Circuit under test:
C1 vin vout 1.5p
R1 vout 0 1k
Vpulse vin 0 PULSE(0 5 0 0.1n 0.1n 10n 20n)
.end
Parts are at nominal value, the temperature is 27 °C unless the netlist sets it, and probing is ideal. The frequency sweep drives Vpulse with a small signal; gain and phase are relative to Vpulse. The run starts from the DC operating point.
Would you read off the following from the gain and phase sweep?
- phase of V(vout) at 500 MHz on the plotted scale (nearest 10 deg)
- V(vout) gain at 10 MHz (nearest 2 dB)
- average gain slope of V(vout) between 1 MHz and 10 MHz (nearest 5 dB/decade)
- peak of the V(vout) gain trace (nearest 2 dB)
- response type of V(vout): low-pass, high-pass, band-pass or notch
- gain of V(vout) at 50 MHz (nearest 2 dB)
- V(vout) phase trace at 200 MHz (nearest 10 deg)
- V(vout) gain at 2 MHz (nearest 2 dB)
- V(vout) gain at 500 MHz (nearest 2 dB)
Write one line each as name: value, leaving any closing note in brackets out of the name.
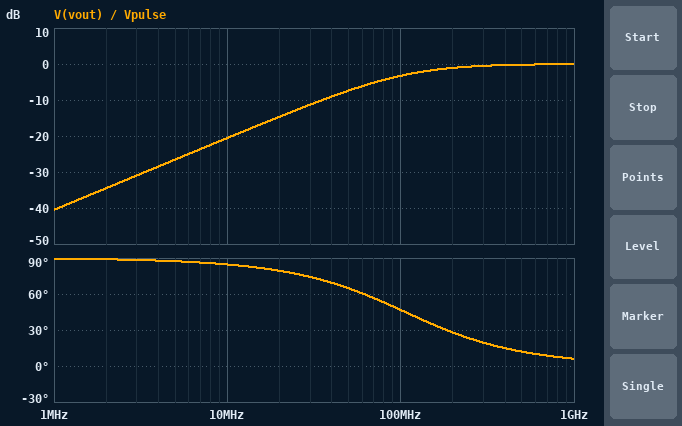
phase of V(vout) at 500 MHz on the plotted scale: 10 deg
V(vout) gain at 10 MHz: -20 dB
average gain slope of V(vout) between 1 MHz and 10 MHz: 20 dB/decade
peak of the V(vout) gain trace: 0 dB
response type of V(vout): low-pass, high-pass, band-pass or notch: high-pass
gain of V(vout) at 50 MHz: -8 dB
V(vout) phase trace at 200 MHz: 30 deg
V(vout) gain at 2 MHz: -34 dB
V(vout) gain at 500 MHz: 0 dB
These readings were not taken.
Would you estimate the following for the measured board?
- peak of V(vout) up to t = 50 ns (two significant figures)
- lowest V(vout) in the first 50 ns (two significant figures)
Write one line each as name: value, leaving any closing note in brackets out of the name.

peak of V(vout) up to t = 50 ns: 4.8 V
lowest V(vout) in the first 50 ns: -4.8 V
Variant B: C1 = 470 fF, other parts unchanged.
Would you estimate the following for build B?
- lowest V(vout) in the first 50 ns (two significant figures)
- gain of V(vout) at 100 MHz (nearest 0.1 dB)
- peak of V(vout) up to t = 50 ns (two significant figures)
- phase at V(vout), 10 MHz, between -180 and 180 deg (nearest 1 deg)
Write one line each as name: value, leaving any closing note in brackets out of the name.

lowest V(vout) in the first 50 ns: -4.5 V
gain of V(vout) at 100 MHz: -11.0 dB
peak of V(vout) up to t = 50 ns: 4.5 V
phase at V(vout), 10 MHz, between -180 and 180 deg: 88 deg
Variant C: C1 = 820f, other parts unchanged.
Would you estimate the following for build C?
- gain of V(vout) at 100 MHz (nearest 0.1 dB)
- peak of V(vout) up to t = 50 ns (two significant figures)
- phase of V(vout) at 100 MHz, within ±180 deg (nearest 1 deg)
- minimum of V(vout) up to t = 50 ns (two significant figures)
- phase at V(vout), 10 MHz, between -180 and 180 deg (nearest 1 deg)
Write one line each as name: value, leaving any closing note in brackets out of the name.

gain of V(vout) at 100 MHz: -6.8 dB
peak of V(vout) up to t = 50 ns: 4.7 V
phase of V(vout) at 100 MHz, within ±180 deg: 63 deg
minimum of V(vout) up to t = 50 ns: -4.7 V
phase at V(vout), 10 MHz, between -180 and 180 deg: 87 deg
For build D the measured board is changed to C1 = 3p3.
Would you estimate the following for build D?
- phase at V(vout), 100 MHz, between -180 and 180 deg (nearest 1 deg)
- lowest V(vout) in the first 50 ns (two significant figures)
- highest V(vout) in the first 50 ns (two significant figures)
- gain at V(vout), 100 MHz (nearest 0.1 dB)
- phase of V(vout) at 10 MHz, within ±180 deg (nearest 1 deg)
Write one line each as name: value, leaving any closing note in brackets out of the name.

phase at V(vout), 100 MHz, between -180 and 180 deg: 26 deg
lowest V(vout) in the first 50 ns: -4.7 V
highest V(vout) in the first 50 ns: 4.9 V
gain at V(vout), 100 MHz: -0.9 dB
phase of V(vout) at 10 MHz, within ±180 deg: 78 deg
